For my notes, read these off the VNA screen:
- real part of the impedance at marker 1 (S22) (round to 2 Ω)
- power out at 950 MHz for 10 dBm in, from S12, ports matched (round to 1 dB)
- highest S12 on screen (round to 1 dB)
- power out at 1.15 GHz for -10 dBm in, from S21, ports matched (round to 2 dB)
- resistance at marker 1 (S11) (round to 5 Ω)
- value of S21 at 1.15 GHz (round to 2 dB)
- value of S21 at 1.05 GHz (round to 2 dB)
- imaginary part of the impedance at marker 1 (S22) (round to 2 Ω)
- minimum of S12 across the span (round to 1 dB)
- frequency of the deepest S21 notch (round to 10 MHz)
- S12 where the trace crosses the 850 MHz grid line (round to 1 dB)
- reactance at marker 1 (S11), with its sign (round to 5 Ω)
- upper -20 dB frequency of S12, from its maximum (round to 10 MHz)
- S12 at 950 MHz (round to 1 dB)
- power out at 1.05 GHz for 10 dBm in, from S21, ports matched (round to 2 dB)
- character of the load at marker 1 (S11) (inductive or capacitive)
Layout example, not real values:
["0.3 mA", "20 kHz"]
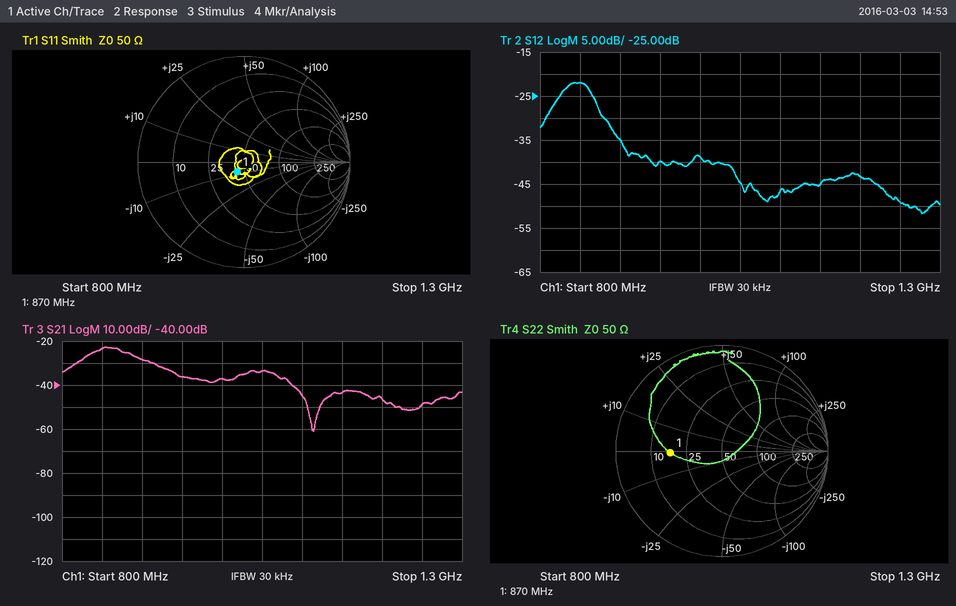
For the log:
["18 Ω", "-30 dBm", "-22 dB", "-54 dBm", "45 Ω", "-44 dB", "-34 dB", "0 Ω", "-52 dB", "1.11 GHz", "-22 dB", "-10 Ω", "1.04 GHz", "-40 dB", "-24 dBm", "capacitive"]
